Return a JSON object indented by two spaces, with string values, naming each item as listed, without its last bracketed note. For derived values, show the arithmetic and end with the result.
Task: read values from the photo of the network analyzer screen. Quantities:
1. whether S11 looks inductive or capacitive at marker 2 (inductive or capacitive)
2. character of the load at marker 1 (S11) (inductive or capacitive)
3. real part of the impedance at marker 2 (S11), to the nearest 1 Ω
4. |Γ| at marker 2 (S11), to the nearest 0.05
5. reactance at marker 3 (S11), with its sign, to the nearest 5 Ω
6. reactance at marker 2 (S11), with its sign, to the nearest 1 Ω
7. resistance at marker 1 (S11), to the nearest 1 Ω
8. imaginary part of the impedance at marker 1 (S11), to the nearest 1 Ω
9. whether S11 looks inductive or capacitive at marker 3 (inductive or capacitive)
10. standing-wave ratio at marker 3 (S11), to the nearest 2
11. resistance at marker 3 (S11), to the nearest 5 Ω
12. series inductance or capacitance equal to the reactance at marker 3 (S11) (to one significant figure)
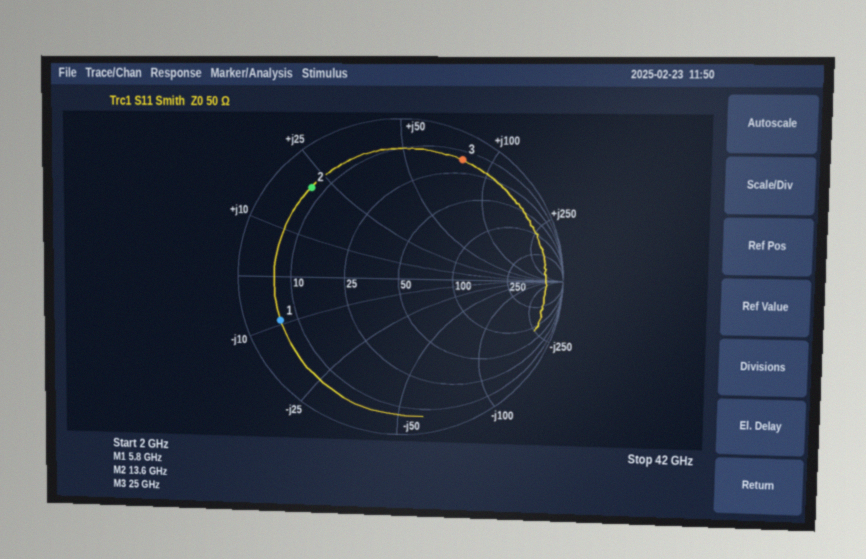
{
  "whether S11 looks inductive or capacitive at marker 2": "inductive",
  "character of the load at marker 1 (S11)": "capacitive",
  "real part of the impedance at marker 2 (S11), to the nearest 1 Ω": "7 Ω",
  "|Γ| at marker 2 (S11), to the nearest 0.05": "0.80",
  "reactance at marker 3 (S11), with its sign, to the nearest 5 Ω": "+80 Ω",
  "reactance at marker 2 (S11), with its sign, to the nearest 1 Ω": "+21 Ω",
  "resistance at marker 1 (S11), to the nearest 1 Ω": "6 Ω",
  "imaginary part of the impedance at marker 1 (S11), to the nearest 1 Ω": "-9 Ω",
  "whether S11 looks inductive or capacitive at marker 3": "inductive",
  "standing-wave ratio at marker 3 (S11), to the nearest 2": "12",
  "resistance at marker 3 (S11), to the nearest 5 Ω": "15 Ω",
  "series inductance or capacitance equal to the reactance at marker 3 (S11)": "L = 80 Ω/(2π × 25 GHz) ≈ 509 pH, so 500 pH to one significant figure"
}
